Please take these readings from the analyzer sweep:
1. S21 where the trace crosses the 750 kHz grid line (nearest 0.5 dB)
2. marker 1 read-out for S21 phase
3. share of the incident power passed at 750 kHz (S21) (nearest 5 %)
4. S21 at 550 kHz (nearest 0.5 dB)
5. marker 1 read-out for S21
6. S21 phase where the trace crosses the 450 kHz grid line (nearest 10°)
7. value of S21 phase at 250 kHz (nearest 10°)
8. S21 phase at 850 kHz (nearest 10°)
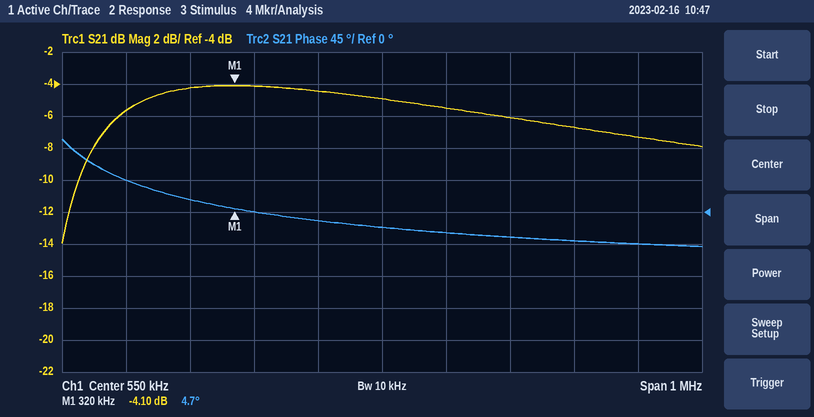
-6.0 dB
4.7°
25 %
-5.0 dB
-4.10 dB
-10°
20°
-40°
